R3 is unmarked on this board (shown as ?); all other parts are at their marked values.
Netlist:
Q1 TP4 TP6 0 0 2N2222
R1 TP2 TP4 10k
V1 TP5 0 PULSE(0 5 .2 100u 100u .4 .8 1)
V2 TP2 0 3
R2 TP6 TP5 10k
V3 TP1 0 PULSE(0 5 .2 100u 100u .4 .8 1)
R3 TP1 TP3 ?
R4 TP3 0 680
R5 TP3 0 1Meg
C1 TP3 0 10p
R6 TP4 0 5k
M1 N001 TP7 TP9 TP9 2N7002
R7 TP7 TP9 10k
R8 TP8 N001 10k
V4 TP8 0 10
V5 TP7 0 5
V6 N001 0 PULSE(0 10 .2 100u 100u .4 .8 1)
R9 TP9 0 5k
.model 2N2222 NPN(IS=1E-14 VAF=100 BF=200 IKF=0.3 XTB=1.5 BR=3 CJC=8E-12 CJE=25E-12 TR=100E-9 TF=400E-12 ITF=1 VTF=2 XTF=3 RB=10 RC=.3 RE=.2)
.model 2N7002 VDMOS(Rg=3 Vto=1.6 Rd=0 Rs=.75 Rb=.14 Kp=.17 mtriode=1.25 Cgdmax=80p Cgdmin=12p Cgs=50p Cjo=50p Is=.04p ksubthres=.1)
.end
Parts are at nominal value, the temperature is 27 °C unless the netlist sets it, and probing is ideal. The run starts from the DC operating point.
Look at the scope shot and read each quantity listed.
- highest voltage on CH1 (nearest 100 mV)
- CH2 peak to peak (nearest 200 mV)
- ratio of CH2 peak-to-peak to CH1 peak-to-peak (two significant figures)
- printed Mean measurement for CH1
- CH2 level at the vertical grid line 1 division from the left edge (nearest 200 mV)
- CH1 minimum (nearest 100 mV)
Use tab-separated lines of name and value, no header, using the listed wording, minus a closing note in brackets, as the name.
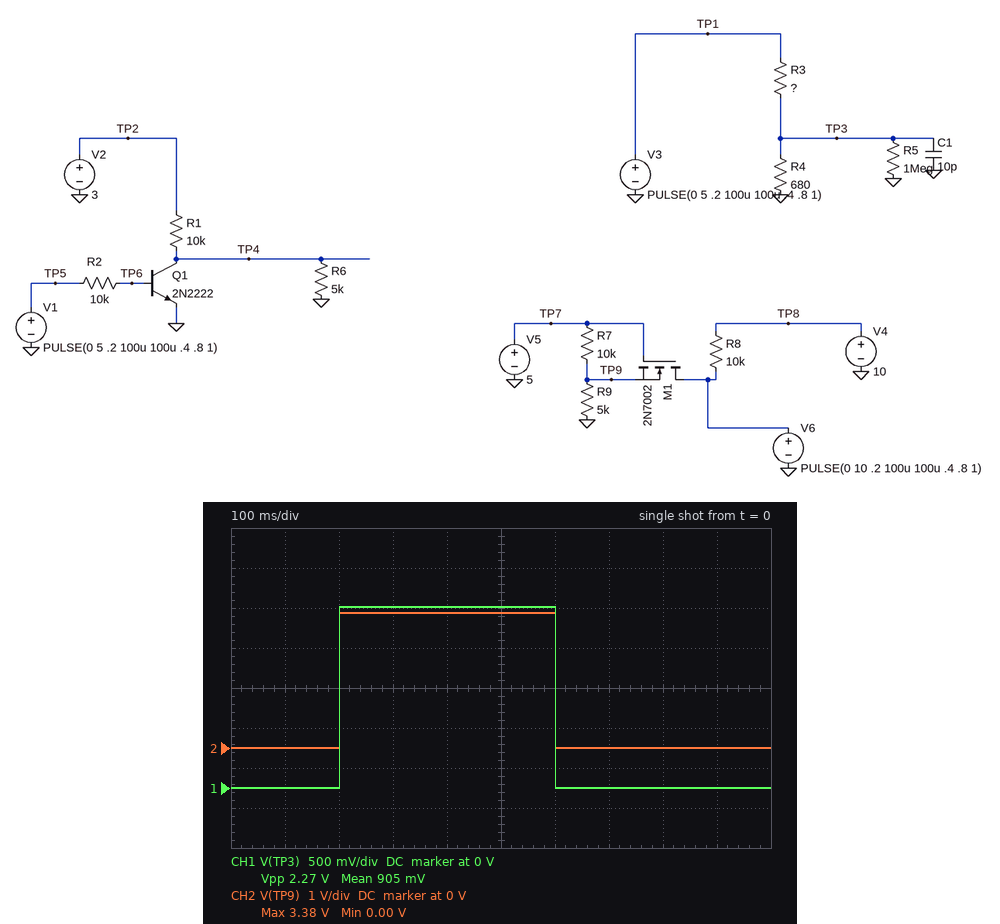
highest voltage on CH1	2.3 V
CH2 peak to peak	3.4 V
ratio of CH2 peak-to-peak to CH1 peak-to-peak	1.5
printed Mean measurement for CH1	905 mV
CH2 level at the vertical grid line 1 division from the left edge	0 V
CH1 minimum	0 V
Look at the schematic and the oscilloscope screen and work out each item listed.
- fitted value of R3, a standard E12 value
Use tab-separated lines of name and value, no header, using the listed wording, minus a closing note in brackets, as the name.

fitted value of R3, a standard E12 value	820 Ω
